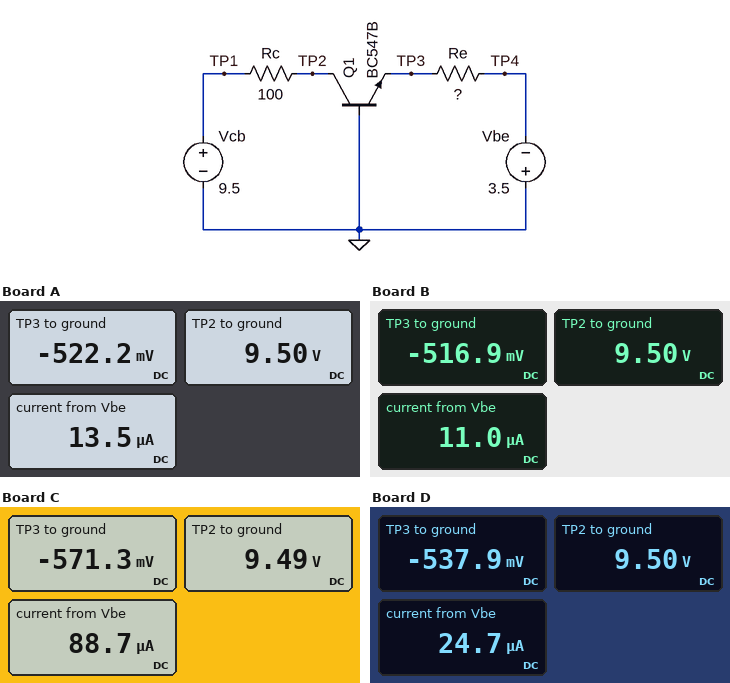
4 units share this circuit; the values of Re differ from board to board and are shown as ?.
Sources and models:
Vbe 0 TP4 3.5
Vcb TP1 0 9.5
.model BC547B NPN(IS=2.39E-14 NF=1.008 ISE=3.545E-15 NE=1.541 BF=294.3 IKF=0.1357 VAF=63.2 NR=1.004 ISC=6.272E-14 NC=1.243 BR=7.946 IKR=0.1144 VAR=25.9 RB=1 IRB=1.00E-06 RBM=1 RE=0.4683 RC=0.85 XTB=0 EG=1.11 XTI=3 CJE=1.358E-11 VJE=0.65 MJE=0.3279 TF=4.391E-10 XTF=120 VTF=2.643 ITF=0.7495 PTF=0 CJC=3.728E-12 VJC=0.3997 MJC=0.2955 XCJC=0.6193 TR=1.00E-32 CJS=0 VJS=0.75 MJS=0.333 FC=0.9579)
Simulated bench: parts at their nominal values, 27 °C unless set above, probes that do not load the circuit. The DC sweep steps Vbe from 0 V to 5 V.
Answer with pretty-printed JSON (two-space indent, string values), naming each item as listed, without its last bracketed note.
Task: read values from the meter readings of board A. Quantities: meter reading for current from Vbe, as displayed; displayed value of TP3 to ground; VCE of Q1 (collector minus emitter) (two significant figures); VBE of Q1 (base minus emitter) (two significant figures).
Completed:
{
  "meter reading for current from Vbe, as displayed": "13.5 µA",
  "displayed value of TP3 to ground": "-522.2 mV",
  "VCE of Q1 (collector minus emitter)": "10 V",
  "VBE of Q1 (base minus emitter)": "520 mV"
}
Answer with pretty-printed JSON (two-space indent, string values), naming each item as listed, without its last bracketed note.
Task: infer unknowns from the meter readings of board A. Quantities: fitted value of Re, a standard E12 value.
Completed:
{
  "fitted value of Re, a standard E12 value": "220 kΩ"
}
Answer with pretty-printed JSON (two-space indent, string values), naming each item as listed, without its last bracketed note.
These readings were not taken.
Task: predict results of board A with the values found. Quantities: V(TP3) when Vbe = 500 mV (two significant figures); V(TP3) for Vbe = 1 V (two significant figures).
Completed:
{
  "V(TP3) when Vbe = 500 mV": "-430 mV",
  "V(TP3) for Vbe = 1 V": "-480 mV"
}
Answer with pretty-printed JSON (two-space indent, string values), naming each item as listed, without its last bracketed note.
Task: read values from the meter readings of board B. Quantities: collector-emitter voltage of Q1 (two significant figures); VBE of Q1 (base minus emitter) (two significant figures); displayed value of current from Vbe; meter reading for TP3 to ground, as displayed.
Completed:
{
  "collector-emitter voltage of Q1": "10 V",
  "VBE of Q1 (base minus emitter)": "520 mV",
  "displayed value of current from Vbe": "11.0 µA",
  "meter reading for TP3 to ground, as displayed": "-516.9 mV"
}
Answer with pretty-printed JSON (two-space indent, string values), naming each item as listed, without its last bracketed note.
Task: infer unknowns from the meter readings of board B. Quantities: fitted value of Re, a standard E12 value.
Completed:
{
  "fitted value of Re, a standard E12 value": "270 kΩ"
}
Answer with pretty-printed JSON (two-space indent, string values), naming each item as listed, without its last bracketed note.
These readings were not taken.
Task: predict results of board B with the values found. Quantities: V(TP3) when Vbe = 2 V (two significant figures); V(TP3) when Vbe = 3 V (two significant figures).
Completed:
{
  "V(TP3) when Vbe = 2 V": "-500 mV",
  "V(TP3) when Vbe = 3 V": "-510 mV"
}
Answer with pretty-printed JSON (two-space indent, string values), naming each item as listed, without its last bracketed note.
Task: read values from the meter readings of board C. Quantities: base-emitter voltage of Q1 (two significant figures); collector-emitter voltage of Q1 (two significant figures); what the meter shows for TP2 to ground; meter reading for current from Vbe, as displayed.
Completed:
{
  "base-emitter voltage of Q1": "570 mV",
  "collector-emitter voltage of Q1": "10 V",
  "what the meter shows for TP2 to ground": "9.49 V",
  "meter reading for current from Vbe, as displayed": "88.7 µA"
}
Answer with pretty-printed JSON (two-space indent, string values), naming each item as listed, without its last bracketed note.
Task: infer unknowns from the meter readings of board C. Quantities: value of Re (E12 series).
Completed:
{
  "value of Re": "33 kΩ"
}
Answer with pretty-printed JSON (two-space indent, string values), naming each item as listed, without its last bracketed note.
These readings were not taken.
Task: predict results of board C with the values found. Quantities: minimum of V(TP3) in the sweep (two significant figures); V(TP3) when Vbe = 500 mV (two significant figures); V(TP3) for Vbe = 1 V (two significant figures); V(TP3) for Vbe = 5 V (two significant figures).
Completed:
{
  "minimum of V(TP3) in the sweep": "-580 mV",
  "V(TP3) when Vbe = 500 mV": "-460 mV",
  "V(TP3) for Vbe = 1 V": "-520 mV",
  "V(TP3) for Vbe = 5 V": "-580 mV"
}
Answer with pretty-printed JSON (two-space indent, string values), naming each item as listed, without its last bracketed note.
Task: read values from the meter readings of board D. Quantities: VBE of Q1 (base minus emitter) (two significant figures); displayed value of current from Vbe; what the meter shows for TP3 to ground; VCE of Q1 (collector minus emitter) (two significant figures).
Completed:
{
  "VBE of Q1 (base minus emitter)": "540 mV",
  "displayed value of current from Vbe": "24.7 µA",
  "what the meter shows for TP3 to ground": "-537.9 mV",
  "VCE of Q1 (collector minus emitter)": "10 V"
}
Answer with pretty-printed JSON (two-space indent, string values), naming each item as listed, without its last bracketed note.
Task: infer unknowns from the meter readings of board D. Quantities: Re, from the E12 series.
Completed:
{
  "Re, from the E12 series": "120 kΩ"
}
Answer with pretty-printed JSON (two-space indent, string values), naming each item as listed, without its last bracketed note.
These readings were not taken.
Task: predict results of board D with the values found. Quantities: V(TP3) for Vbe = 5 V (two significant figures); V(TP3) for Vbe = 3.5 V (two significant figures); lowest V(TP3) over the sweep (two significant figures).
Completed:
{
  "V(TP3) for Vbe = 5 V": "-550 mV",
  "V(TP3) for Vbe = 3.5 V": "-540 mV",
  "lowest V(TP3) over the sweep": "-550 mV"
}
